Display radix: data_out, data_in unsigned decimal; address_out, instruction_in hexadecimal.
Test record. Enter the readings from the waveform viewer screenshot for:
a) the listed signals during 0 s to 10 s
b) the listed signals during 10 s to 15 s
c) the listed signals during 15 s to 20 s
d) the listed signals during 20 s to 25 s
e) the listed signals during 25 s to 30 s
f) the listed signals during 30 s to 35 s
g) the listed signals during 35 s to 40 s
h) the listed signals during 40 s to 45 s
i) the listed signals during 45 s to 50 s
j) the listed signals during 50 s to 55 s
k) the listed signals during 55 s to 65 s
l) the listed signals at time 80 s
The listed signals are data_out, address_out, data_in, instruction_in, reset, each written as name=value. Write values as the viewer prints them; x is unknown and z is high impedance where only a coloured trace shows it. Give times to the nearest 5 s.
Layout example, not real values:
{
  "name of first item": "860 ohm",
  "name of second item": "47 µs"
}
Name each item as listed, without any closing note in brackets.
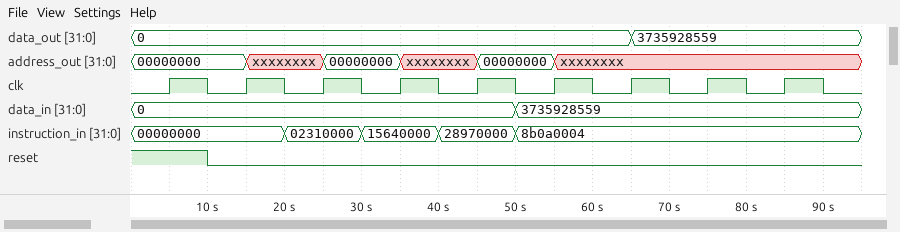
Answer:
{
  "the listed signals during 0 s to 10 s": "data_out=0, address_out=00000000, data_in=0, instruction_in=00000000, reset=1",
  "the listed signals during 10 s to 15 s": "data_out=0, address_out=00000000, data_in=0, instruction_in=00000000, reset=0",
  "the listed signals during 15 s to 20 s": "data_out=0, address_out=xxxxxxxx, data_in=0, instruction_in=00000000, reset=0",
  "the listed signals during 20 s to 25 s": "data_out=0, address_out=xxxxxxxx, data_in=0, instruction_in=02310000, reset=0",
  "the listed signals during 25 s to 30 s": "data_out=0, address_out=00000000, data_in=0, instruction_in=02310000, reset=0",
  "the listed signals during 30 s to 35 s": "data_out=0, address_out=00000000, data_in=0, instruction_in=15640000, reset=0",
  "the listed signals during 35 s to 40 s": "data_out=0, address_out=xxxxxxxx, data_in=0, instruction_in=15640000, reset=0",
  "the listed signals during 40 s to 45 s": "data_out=0, address_out=xxxxxxxx, data_in=0, instruction_in=28970000, reset=0",
  "the listed signals during 45 s to 50 s": "data_out=0, address_out=00000000, data_in=0, instruction_in=28970000, reset=0",
  "the listed signals during 50 s to 55 s": "data_out=0, address_out=00000000, data_in=3735928559, instruction_in=8b0a0004, reset=0",
  "the listed signals during 55 s to 65 s": "data_out=0, address_out=xxxxxxxx, data_in=3735928559, instruction_in=8b0a0004, reset=0",
  "the listed signals at time 80 s": "data_out=3735928559, address_out=xxxxxxxx, data_in=3735928559, instruction_in=8b0a0004, reset=0"
}
